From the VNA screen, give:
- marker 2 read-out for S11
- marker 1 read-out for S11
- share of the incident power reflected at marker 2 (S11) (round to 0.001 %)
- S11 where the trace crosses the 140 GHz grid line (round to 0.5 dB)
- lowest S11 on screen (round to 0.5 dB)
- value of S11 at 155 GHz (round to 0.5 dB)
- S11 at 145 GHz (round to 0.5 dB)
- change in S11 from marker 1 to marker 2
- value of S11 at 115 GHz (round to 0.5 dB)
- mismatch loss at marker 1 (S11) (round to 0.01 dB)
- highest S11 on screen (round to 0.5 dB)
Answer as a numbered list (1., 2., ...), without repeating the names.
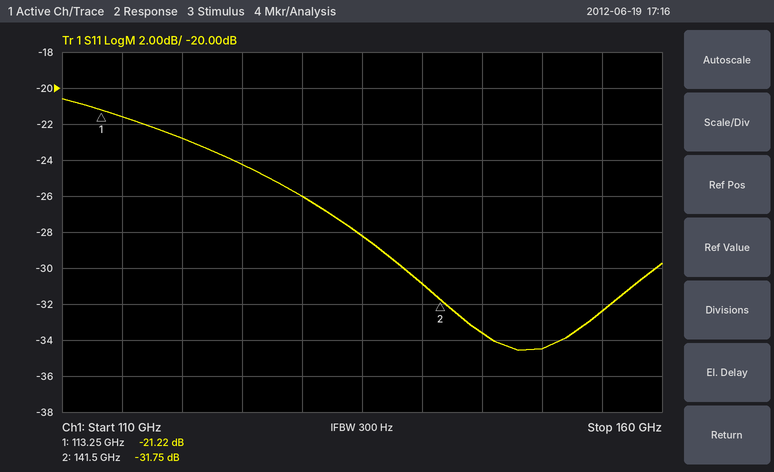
1. -31.75 dB
2. -21.22 dB
3. 0.067 %
4. -31.0 dB
5. -34.5 dB
6. -32.5 dB
7. -33.5 dB
8. -10.53 dB
9. -21.5 dB
10. 0.03 dB
11. -20.5 dB
